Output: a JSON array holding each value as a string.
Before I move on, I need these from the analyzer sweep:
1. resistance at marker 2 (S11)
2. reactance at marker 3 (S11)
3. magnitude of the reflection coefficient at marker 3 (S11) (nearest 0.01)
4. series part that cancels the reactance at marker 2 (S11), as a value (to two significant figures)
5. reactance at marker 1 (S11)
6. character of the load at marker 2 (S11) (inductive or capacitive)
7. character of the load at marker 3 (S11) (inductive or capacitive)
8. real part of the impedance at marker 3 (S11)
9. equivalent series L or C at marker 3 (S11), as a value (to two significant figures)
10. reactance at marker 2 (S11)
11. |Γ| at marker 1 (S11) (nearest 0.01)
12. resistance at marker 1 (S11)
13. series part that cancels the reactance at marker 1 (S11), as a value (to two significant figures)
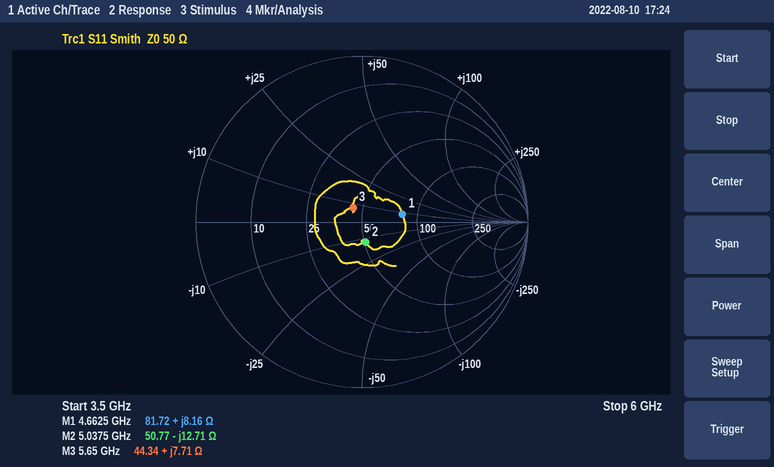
["50.77 Ω", "+7.71 Ω", "0.10", "400 pH", "+8.16 Ω", "capacitive", "inductive", "44.34 Ω", "220 pH", "-12.71 Ω", "0.25", "81.72 Ω", "4.2 pF"]
